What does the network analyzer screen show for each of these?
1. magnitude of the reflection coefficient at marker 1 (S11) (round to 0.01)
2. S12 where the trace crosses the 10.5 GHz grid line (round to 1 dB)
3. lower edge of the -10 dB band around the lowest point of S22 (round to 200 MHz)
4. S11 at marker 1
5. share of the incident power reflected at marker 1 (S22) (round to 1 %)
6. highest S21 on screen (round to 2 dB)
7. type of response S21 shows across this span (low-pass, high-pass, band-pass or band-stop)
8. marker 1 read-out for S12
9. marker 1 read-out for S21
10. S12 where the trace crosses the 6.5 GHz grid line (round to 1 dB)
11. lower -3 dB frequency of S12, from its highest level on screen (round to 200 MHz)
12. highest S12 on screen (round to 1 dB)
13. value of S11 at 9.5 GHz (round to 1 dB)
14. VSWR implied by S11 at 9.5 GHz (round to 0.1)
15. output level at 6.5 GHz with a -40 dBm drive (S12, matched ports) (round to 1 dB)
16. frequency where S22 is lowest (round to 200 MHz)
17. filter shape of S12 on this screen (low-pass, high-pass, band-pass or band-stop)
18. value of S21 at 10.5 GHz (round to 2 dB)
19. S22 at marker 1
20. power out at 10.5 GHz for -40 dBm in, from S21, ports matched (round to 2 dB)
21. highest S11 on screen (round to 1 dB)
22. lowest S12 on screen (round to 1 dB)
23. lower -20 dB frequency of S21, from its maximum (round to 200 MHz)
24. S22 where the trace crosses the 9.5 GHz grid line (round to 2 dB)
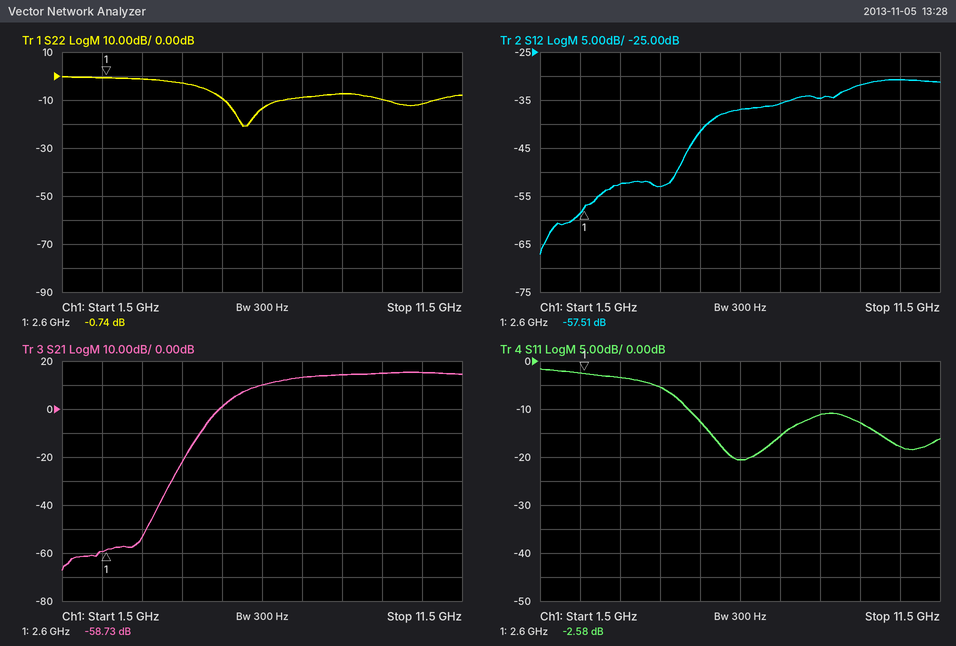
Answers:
0.74
-31 dB
5.6 GHz
-2.58 dB
84 %
16 dB
high-pass
-57.51 dB
-58.73 dB
-37 dB
9.0 GHz
-31 dB
-13 dB
1.6
-77 dBm
6.0 GHz
high-pass
16 dB
-0.74 dB
-24 dBm
-2 dB
-67 dB
5.2 GHz
-10 dB
